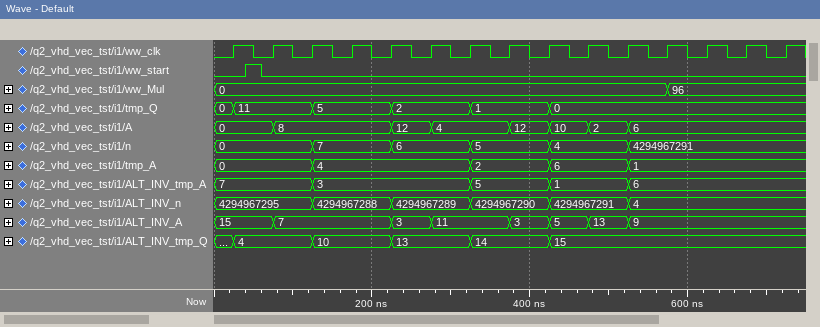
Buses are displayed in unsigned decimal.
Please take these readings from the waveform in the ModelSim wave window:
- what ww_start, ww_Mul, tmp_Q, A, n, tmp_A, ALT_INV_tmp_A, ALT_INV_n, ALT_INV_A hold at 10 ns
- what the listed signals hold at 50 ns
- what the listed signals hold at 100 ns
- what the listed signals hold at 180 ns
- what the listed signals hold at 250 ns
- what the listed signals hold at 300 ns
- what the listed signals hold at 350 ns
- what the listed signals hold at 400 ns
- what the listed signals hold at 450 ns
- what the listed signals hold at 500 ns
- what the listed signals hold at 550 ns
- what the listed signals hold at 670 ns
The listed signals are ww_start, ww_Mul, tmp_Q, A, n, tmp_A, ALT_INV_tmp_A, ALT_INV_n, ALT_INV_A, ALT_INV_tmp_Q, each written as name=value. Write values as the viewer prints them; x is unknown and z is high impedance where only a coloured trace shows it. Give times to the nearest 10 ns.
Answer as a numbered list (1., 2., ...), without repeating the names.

1. ww_start=0, ww_Mul=0, tmp_Q=0, A=0, n=0, tmp_A=0, ALT_INV_tmp_A=7, ALT_INV_n=4294967295, ALT_INV_A=15
2. ww_start=1, ww_Mul=0, tmp_Q=11, A=0, n=0, tmp_A=0, ALT_INV_tmp_A=7, ALT_INV_n=4294967295, ALT_INV_A=15, ALT_INV_tmp_Q=4
3. ww_start=0, ww_Mul=0, tmp_Q=11, A=8, n=0, tmp_A=0, ALT_INV_tmp_A=7, ALT_INV_n=4294967295, ALT_INV_A=7, ALT_INV_tmp_Q=4
4. ww_start=0, ww_Mul=0, tmp_Q=5, A=8, n=7, tmp_A=4, ALT_INV_tmp_A=3, ALT_INV_n=4294967288, ALT_INV_A=7, ALT_INV_tmp_Q=10
5. ww_start=0, ww_Mul=0, tmp_Q=2, A=12, n=6, tmp_A=4, ALT_INV_tmp_A=3, ALT_INV_n=4294967289, ALT_INV_A=3, ALT_INV_tmp_Q=13
6. ww_start=0, ww_Mul=0, tmp_Q=2, A=4, n=6, tmp_A=4, ALT_INV_tmp_A=3, ALT_INV_n=4294967289, ALT_INV_A=11, ALT_INV_tmp_Q=13
7. ww_start=0, ww_Mul=0, tmp_Q=1, A=4, n=5, tmp_A=2, ALT_INV_tmp_A=5, ALT_INV_n=4294967290, ALT_INV_A=11, ALT_INV_tmp_Q=14
8. ww_start=0, ww_Mul=0, tmp_Q=1, A=12, n=5, tmp_A=2, ALT_INV_tmp_A=5, ALT_INV_n=4294967290, ALT_INV_A=3, ALT_INV_tmp_Q=14
9. ww_start=0, ww_Mul=0, tmp_Q=0, A=10, n=4, tmp_A=6, ALT_INV_tmp_A=1, ALT_INV_n=4294967291, ALT_INV_A=5, ALT_INV_tmp_Q=15
10. ww_start=0, ww_Mul=0, tmp_Q=0, A=2, n=4, tmp_A=6, ALT_INV_tmp_A=1, ALT_INV_n=4294967291, ALT_INV_A=13, ALT_INV_tmp_Q=15
11. ww_start=0, ww_Mul=0, tmp_Q=0, A=6, n=4294967291, tmp_A=1, ALT_INV_tmp_A=6, ALT_INV_n=4, ALT_INV_A=9, ALT_INV_tmp_Q=15
12. ww_start=0, ww_Mul=96, tmp_Q=0, A=6, n=4294967291, tmp_A=1, ALT_INV_tmp_A=6, ALT_INV_n=4, ALT_INV_A=9, ALT_INV_tmp_Q=15
